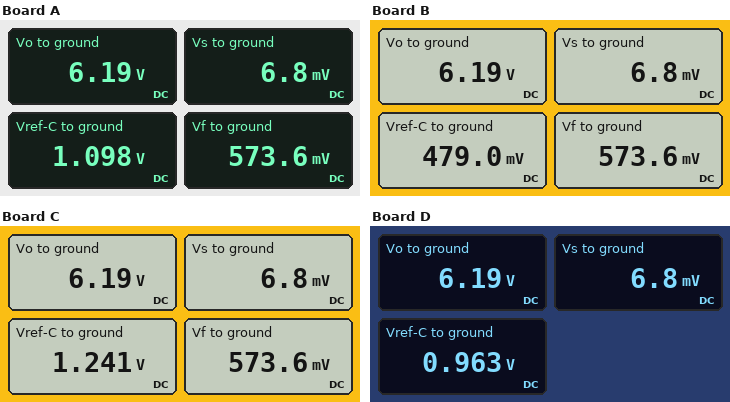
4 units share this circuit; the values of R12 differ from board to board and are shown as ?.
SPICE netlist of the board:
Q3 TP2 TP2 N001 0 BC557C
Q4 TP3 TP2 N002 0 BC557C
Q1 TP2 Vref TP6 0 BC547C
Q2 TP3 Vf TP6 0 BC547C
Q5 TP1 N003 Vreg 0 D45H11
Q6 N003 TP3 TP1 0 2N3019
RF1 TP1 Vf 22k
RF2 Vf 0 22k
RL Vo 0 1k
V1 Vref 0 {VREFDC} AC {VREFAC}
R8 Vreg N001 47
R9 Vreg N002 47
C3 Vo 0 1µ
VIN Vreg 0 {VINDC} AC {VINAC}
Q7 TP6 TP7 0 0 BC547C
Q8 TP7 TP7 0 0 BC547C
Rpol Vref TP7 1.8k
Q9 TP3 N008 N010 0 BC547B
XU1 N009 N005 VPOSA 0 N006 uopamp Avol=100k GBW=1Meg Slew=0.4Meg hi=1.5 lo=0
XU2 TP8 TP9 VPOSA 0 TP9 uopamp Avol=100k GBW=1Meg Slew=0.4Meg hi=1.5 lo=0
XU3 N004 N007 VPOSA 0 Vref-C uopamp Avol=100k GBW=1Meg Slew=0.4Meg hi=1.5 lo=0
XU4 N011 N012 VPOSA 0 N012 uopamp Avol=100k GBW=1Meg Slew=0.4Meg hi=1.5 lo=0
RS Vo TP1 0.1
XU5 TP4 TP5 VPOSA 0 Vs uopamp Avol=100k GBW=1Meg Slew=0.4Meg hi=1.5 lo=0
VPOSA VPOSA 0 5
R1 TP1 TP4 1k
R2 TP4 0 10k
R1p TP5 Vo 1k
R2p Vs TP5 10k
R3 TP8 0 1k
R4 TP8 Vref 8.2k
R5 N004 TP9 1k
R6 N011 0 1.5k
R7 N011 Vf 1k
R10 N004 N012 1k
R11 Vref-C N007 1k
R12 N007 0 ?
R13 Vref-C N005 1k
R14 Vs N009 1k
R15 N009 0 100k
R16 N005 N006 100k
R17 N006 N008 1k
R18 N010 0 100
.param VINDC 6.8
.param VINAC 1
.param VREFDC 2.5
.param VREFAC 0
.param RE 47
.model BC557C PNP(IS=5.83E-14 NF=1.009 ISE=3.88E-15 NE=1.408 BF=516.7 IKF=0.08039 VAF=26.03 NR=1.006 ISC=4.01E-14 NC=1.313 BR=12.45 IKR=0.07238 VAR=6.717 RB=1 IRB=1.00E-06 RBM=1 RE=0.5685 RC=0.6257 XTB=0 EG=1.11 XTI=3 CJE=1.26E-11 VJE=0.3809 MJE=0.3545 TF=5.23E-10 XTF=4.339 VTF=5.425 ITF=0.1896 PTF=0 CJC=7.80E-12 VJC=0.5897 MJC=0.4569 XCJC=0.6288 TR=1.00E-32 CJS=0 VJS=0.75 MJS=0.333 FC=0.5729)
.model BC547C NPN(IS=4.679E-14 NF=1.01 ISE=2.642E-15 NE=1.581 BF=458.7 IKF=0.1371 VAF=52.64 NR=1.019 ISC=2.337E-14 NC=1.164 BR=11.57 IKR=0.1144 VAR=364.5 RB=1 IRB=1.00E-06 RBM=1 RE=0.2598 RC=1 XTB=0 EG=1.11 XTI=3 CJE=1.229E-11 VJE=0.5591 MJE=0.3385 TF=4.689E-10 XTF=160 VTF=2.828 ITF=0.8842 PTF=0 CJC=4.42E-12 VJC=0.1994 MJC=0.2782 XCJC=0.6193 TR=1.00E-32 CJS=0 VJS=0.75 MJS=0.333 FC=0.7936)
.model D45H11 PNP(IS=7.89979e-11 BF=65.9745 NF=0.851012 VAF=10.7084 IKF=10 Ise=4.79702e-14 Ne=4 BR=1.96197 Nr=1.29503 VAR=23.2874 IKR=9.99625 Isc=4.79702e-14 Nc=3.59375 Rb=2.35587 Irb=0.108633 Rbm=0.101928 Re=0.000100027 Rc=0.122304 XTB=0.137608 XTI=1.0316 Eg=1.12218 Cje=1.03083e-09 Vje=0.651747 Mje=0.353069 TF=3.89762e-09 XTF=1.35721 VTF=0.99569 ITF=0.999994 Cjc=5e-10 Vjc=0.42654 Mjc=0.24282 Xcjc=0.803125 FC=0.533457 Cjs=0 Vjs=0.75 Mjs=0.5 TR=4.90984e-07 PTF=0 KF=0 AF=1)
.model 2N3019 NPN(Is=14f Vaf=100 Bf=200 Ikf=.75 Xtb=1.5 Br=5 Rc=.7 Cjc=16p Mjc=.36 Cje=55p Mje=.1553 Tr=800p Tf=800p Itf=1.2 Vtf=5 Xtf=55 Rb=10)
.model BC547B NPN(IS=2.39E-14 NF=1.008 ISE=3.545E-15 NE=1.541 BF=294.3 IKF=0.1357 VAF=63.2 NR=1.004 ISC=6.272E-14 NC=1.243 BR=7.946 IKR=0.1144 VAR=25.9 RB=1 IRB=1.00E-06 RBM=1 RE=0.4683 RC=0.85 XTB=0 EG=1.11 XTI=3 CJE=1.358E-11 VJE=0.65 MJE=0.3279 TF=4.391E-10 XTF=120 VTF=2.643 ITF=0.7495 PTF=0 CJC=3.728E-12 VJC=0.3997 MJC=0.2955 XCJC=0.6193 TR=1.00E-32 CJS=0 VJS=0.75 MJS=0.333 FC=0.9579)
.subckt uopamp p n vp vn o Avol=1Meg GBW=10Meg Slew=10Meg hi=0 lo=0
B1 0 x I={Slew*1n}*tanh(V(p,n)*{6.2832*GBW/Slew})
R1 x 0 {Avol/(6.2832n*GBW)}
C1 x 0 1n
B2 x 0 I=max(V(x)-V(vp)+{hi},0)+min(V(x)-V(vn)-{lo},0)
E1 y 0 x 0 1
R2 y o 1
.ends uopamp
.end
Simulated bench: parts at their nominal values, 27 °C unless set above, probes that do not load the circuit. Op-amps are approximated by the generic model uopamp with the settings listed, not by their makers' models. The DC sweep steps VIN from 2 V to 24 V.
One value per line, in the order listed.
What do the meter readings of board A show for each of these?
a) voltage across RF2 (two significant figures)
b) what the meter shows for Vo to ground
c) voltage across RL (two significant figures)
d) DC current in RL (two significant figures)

570 mV
6.19 V
6.2 V
6.2 mA
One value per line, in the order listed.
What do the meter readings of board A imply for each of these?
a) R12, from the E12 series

390 Ω
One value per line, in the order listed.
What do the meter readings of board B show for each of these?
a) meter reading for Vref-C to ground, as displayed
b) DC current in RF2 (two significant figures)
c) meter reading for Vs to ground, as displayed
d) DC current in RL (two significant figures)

479.0 mV
26 µA
6.8 mV
6.2 mA
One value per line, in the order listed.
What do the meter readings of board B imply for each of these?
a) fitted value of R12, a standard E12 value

1.8 kΩ
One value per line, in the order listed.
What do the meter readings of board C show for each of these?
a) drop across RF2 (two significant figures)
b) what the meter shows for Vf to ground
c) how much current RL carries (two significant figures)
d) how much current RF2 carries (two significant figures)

570 mV
573.6 mV
6.2 mA
26 µA
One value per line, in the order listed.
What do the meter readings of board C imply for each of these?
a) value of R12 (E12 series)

330 Ω
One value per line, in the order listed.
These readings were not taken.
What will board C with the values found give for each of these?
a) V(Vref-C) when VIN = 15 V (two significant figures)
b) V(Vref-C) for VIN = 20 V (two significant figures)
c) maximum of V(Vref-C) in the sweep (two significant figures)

2.2 V
2.7 V
3.2 V
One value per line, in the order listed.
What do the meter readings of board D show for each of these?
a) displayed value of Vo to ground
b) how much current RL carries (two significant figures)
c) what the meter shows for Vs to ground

6.19 V
6.2 mA
6.8 mV
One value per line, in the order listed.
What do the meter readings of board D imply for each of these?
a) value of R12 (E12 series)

470 Ω
